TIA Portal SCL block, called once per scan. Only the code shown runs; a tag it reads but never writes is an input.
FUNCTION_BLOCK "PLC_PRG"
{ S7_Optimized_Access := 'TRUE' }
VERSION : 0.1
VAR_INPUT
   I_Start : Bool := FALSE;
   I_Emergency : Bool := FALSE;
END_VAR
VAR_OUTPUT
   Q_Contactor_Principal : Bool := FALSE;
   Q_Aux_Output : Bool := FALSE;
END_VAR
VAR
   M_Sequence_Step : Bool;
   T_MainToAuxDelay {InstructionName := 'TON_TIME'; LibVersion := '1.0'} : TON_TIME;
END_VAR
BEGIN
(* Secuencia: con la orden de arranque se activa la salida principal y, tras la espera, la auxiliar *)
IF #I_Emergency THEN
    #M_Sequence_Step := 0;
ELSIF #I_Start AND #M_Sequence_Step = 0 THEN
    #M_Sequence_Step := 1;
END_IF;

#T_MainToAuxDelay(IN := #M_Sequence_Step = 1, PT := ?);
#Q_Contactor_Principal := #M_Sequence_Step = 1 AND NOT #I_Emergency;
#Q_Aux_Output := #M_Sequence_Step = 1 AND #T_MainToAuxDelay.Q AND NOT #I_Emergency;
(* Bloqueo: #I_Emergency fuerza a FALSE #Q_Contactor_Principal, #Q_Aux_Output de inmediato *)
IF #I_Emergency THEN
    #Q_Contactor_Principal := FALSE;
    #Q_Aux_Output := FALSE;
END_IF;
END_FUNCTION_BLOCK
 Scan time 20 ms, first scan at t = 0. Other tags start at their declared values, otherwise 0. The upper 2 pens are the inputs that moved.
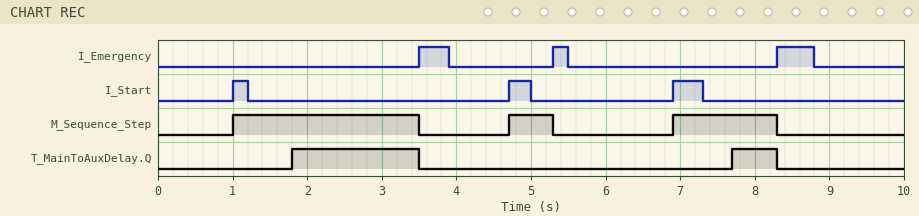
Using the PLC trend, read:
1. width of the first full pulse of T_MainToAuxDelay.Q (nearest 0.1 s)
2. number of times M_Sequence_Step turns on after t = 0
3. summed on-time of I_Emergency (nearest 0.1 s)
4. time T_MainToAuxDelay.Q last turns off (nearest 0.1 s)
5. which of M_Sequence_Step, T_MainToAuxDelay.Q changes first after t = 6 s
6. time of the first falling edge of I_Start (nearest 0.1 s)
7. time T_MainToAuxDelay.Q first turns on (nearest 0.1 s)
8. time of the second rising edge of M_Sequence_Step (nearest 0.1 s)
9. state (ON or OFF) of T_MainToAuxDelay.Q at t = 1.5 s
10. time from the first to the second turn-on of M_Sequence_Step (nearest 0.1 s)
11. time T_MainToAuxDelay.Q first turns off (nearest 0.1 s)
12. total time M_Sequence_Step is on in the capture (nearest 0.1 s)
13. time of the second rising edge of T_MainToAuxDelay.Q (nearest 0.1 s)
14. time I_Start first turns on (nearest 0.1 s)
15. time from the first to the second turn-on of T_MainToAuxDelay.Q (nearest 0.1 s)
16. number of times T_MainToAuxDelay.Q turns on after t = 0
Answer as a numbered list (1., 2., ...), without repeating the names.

1. 1.7 s
2. 3
3. 1.1 s
4. 8.3 s
5. M_Sequence_Step
6. 1.2 s
7. 1.8 s
8. 4.7 s
9. OFF
10. 3.7 s
11. 3.5 s
12. 4.5 s
13. 7.7 s
14. 1.0 s
15. 5.9 s
16. 2
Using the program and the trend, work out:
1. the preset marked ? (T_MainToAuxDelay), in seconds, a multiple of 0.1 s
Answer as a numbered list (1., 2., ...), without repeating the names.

1. 0.8 s
